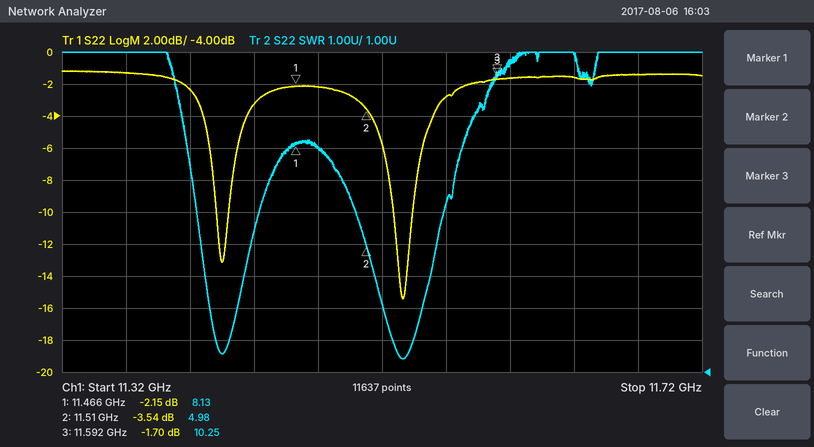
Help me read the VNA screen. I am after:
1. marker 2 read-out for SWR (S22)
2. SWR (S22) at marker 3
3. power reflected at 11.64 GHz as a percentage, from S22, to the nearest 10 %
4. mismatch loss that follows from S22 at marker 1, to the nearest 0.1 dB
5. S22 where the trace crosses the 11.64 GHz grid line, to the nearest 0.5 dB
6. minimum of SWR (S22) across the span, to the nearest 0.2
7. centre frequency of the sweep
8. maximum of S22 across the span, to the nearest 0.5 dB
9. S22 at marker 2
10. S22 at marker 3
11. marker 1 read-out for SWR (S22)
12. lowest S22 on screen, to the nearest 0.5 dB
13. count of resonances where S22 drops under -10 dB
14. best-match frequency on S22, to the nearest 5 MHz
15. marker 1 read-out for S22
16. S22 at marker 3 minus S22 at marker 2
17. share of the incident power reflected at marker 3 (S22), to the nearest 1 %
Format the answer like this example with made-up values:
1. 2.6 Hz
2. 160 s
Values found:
1. 4.98
2. 10.25
3. 70 %
4. 4.1 dB
5. -1.5 dB
6. 1.4
7. 11.52 GHz
8. -1.0 dB
9. -3.54 dB
10. -1.70 dB
11. 8.13
12. -15.5 dB
13. 2
14. 11.535 GHz
15. -2.15 dB
16. 1.84 dB
17. 68 %
